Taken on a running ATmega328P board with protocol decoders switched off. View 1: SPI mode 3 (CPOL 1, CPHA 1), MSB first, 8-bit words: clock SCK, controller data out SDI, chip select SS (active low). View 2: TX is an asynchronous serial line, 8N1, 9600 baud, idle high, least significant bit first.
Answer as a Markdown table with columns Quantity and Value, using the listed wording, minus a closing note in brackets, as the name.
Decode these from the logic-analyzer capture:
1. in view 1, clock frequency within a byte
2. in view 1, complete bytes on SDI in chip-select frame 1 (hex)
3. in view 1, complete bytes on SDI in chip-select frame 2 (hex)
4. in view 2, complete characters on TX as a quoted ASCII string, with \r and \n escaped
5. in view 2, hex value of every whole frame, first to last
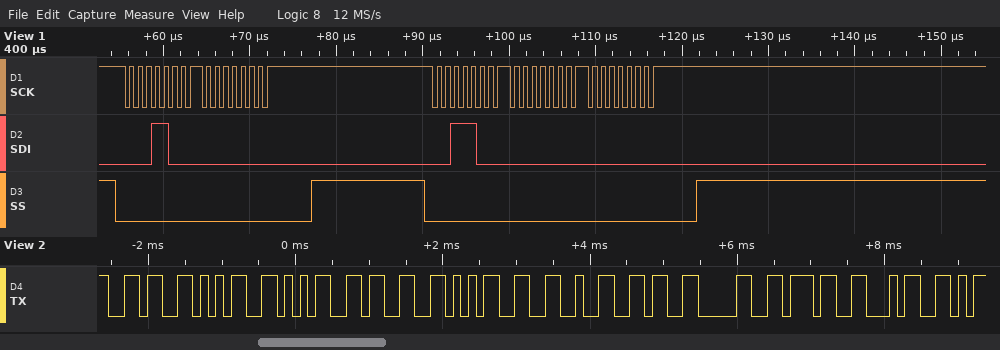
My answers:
| Quantity | Value |
|---|---|
| in view 1, clock frequency within a byte | 1 MHz |
| in view 1, complete bytes on SDI in chip-select frame 1 | 18 00 |
| in view 1, complete bytes on SDI in chip-select frame 2 | 38 00 00 |
| in view 2, complete characters on TX as a quoted ASCII string, with \r and \n escaped | "65535&6074" |
| in view 2, hex value of every whole frame, first to last | 36 35 35 33 35 26 36 30 37 34 |
